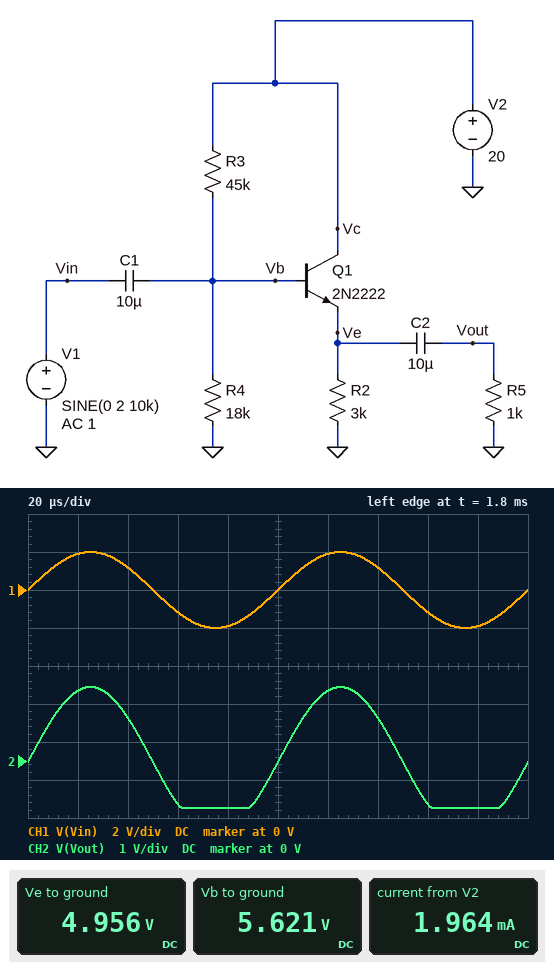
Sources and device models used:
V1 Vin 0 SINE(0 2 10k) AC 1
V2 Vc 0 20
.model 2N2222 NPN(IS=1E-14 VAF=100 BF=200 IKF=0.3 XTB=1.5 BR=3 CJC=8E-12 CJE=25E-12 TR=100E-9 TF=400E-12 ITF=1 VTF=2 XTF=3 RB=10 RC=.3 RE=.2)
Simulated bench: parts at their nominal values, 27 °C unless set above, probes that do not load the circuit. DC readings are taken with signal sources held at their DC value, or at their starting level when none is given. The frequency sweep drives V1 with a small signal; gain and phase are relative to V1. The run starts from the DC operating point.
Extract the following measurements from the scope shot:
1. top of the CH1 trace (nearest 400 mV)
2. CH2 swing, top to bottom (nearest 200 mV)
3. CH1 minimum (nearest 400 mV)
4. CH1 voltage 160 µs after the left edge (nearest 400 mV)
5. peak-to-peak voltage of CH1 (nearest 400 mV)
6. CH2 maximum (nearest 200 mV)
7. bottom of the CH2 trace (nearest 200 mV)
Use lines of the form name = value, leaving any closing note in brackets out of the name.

top of the CH1 trace = 2.0 V
CH2 swing, top to bottom = 3.2 V
CH1 minimum = -2.0 V
CH1 voltage 160 µs after the left edge = -1.2 V
peak-to-peak voltage of CH1 = 4.0 V
CH2 maximum = 2.0 V
bottom of the CH2 trace = -1.2 V
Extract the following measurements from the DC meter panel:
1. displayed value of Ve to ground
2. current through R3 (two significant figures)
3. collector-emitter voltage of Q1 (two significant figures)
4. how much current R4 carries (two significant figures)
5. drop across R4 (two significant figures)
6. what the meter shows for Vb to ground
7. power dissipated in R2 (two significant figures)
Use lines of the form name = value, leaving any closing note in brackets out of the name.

displayed value of Ve to ground = 4.956 V
current through R3 = 320 µA
collector-emitter voltage of Q1 = 15 V
how much current R4 carries = 310 µA
drop across R4 = 5.6 V
what the meter shows for Vb to ground = 5.621 V
power dissipated in R2 = 8.2 mW
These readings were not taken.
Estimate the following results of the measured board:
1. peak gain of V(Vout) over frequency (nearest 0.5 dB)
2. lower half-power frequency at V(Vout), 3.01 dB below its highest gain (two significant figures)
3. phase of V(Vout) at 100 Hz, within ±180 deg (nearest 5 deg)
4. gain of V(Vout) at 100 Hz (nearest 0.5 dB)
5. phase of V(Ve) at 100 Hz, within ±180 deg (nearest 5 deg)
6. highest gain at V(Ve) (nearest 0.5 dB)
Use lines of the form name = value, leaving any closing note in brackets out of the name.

peak gain of V(Vout) over frequency = 0 dB
lower half-power frequency at V(Vout), 3.01 dB below its highest gain = 16 Hz
phase of V(Vout) at 100 Hz, within ±180 deg = 10 deg
gain of V(Vout) at 100 Hz = -0.5 dB
phase of V(Ve) at 100 Hz, within ±180 deg = 0 deg
highest gain at V(Ve) = 0 dB
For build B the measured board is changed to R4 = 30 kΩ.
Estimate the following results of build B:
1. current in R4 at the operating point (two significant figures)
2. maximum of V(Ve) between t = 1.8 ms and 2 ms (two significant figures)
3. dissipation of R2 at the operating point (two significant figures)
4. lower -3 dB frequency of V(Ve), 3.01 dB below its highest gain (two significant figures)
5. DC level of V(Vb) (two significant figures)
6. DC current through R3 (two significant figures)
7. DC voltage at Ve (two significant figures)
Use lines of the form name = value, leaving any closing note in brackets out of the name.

current in R4 at the operating point = 260 µA
maximum of V(Ve) between t = 1.8 ms and 2 ms = 9.1 V
dissipation of R2 at the operating point = 17 mW
lower -3 dB frequency of V(Ve), 3.01 dB below its highest gain = 900 mHz
DC level of V(Vb) = 7.8 V
DC current through R3 = 270 µA
DC voltage at Ve = 7.1 V
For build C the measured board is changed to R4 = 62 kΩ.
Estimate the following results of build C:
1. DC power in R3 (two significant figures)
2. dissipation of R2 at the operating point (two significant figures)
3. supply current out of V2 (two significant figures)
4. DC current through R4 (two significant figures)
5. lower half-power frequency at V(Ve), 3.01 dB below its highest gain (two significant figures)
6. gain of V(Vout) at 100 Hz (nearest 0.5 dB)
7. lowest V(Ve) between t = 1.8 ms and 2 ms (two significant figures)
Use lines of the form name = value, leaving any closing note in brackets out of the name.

DC power in R3 = 1.7 mW
dissipation of R2 at the operating point = 37 mW
supply current out of V2 = 3.7 mA
DC current through R4 = 180 µA
lower half-power frequency at V(Ve), 3.01 dB below its highest gain = 630 mHz
gain of V(Vout) at 100 Hz = 0 dB
lowest V(Ve) between t = 1.8 ms and 2 ms = 8.5 V
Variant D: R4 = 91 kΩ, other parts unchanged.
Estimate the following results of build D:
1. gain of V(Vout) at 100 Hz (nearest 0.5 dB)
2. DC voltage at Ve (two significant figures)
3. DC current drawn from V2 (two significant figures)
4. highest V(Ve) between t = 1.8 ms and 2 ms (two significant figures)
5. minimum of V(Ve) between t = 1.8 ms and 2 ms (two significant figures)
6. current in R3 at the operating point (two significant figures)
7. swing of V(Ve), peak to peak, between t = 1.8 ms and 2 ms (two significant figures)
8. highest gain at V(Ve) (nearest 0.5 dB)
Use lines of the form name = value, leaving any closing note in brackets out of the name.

gain of V(Vout) at 100 Hz = 0 dB
DC voltage at Ve = 12 V
DC current drawn from V2 = 4.2 mA
highest V(Ve) between t = 1.8 ms and 2 ms = 14 V
minimum of V(Ve) between t = 1.8 ms and 2 ms = 10 V
current in R3 at the operating point = 160 µA
swing of V(Ve), peak to peak, between t = 1.8 ms and 2 ms = 4.0 V
highest gain at V(Ve) = 0 dB
